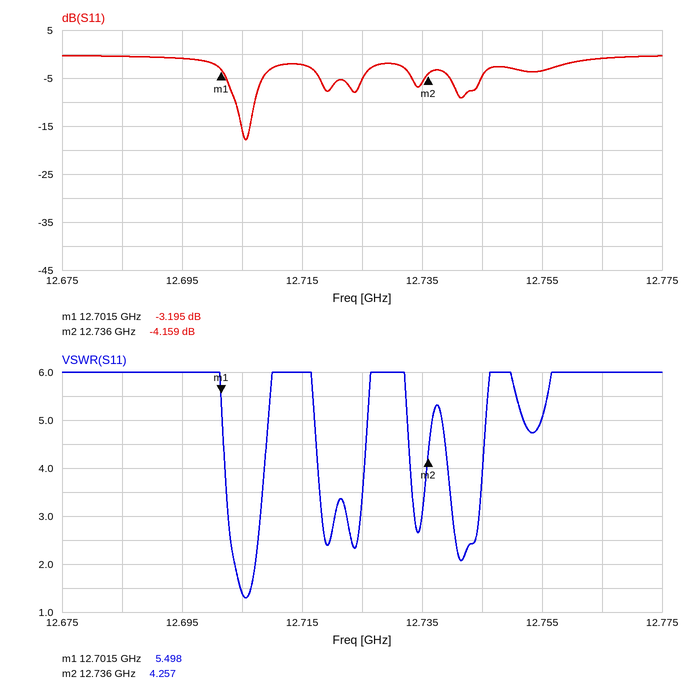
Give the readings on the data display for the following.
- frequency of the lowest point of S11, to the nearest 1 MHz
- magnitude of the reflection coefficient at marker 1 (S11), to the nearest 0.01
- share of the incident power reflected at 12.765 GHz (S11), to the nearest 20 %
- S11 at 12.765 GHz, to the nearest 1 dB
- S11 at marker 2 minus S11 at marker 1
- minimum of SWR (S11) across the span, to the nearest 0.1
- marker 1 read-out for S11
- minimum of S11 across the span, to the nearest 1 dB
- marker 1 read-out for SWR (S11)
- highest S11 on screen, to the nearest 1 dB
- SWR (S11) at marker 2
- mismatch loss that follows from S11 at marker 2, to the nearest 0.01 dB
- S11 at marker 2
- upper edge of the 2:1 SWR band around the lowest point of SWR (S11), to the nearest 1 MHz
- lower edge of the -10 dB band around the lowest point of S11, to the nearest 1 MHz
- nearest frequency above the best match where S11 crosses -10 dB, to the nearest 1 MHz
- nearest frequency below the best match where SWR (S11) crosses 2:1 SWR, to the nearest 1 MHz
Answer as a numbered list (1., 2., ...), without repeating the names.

1. 12.706 GHz
2. 0.69
3. 80 %
4. -1 dB
5. -0.964 dB
6. 1.3
7. -3.195 dB
8. -18 dB
9. 5.498
10. 0 dB
11. 4.257
12. 2.10 dB
13. -4.159 dB
14. 12.707 GHz
15. 12.704 GHz
16. 12.707 GHz
17. 12.704 GHz
